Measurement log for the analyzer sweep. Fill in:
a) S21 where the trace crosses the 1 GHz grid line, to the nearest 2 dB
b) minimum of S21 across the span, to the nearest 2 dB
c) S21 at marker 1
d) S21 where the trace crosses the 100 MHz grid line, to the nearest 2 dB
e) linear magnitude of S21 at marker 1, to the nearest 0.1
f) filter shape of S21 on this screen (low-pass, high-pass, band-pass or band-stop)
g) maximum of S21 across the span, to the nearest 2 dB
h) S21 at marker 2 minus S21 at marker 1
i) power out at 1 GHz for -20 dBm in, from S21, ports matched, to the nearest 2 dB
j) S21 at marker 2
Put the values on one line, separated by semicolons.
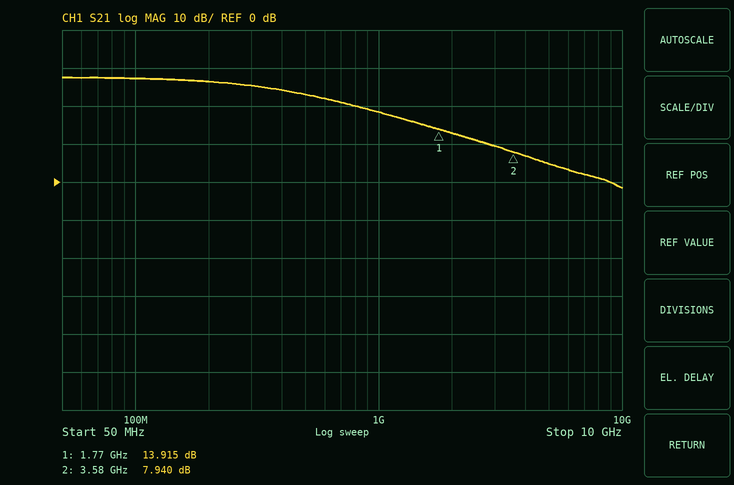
18 dB; -2 dB; 13.915 dB; 28 dB; 5.0; low-pass; 28 dB; -5.975 dB; -2 dBm; 7.940 dB
